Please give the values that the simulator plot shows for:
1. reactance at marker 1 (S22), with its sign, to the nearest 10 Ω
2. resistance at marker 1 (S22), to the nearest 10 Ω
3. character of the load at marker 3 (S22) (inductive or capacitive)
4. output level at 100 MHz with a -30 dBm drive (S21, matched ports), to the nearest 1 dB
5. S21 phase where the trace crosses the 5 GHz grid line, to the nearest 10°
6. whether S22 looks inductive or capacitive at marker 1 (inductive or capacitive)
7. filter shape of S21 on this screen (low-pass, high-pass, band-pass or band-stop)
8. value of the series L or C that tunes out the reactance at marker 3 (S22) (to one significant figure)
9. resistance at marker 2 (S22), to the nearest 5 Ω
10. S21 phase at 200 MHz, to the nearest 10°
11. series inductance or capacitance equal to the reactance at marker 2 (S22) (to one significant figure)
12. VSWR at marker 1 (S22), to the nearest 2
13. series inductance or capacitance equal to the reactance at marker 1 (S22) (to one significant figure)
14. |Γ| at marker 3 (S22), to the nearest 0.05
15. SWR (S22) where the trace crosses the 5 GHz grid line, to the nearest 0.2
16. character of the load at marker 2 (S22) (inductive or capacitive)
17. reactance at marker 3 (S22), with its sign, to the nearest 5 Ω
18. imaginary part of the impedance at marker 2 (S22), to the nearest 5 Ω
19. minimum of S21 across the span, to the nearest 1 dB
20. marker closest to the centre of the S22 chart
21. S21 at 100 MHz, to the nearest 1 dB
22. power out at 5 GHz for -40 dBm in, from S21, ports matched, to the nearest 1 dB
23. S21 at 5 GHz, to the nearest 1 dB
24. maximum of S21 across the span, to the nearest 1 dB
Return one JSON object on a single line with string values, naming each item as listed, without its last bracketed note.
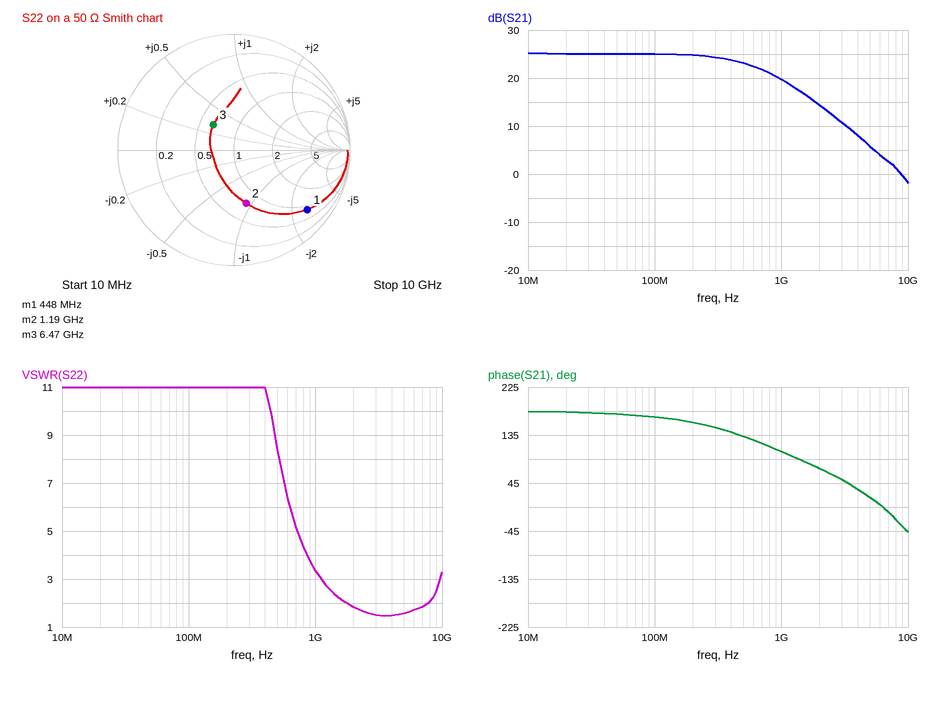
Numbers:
{"reactance at marker 1 (S22), with its sign, to the nearest 10 Ω": "-130 Ω", "resistance at marker 1 (S22), to the nearest 10 Ω": "40 Ω", "character of the load at marker 3 (S22)": "inductive", "output level at 100 MHz with a -30 dBm drive (S21, matched ports), to the nearest 1 dB": "-5 dBm", "S21 phase where the trace crosses the 5 GHz grid line, to the nearest 10°": "20°", "whether S22 looks inductive or capacitive at marker 1": "capacitive", "filter shape of S21 on this screen": "low-pass", "value of the series L or C that tunes out the reactance at marker 3 (S22)": "2 pF", "resistance at marker 2 (S22), to the nearest 5 Ω": "40 Ω", "S21 phase at 200 MHz, to the nearest 10°": "160°", "series inductance or capacitance equal to the reactance at marker 2 (S22)": "3 pF", "VSWR at marker 1 (S22), to the nearest 2": "10", "series inductance or capacitance equal to the reactance at marker 1 (S22)": "3 pF", "|Γ| at marker 3 (S22), to the nearest 0.05": "0.30", "SWR (S22) where the trace crosses the 5 GHz grid line, to the nearest 0.2": "1.6", "character of the load at marker 2 (S22)": "capacitive", "reactance at marker 3 (S22), with its sign, to the nearest 5 Ω": "+15 Ω", "imaginary part of the impedance at marker 2 (S22), to the nearest 5 Ω": "-45 Ω", "minimum of S21 across the span, to the nearest 1 dB": "-2 dB", "marker closest to the centre of the S22 chart": "marker 3", "S21 at 100 MHz, to the nearest 1 dB": "25 dB", "power out at 5 GHz for -40 dBm in, from S21, ports matched, to the nearest 1 dB": "-34 dBm", "S21 at 5 GHz, to the nearest 1 dB": "6 dB", "maximum of S21 across the span, to the nearest 1 dB": "25 dB"}
